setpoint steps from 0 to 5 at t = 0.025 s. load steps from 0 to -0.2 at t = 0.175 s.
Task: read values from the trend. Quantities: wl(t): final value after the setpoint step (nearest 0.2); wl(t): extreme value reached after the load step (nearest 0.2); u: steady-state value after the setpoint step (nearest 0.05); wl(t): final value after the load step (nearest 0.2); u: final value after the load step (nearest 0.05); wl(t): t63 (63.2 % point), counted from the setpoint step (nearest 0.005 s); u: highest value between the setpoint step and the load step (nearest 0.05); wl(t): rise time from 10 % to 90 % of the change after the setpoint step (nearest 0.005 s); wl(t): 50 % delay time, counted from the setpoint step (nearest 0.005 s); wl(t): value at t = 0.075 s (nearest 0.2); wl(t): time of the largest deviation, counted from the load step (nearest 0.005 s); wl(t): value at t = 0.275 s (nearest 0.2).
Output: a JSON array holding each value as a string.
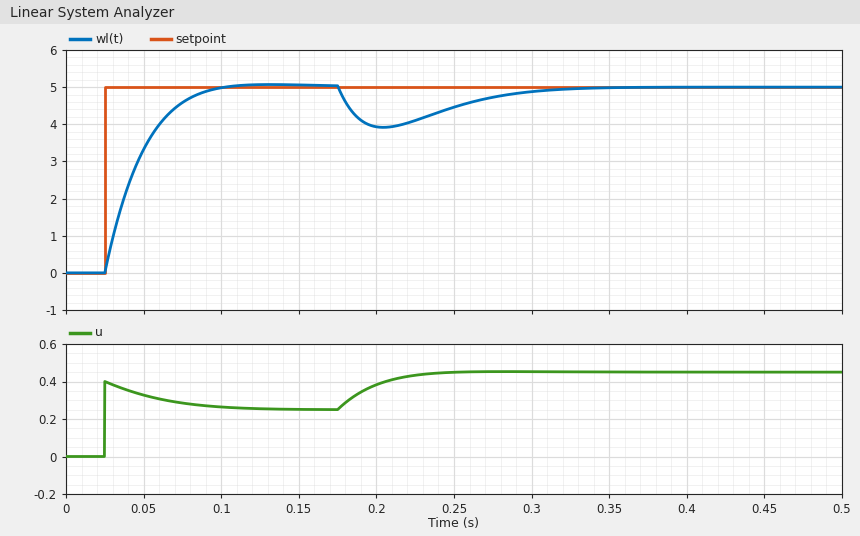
["5.0", "4.0", "0.25", "5.0", "0.45", "0.025 s", "0.40", "0.045 s", "0.015 s", "4.6", "0.030 s", "4.8"]
